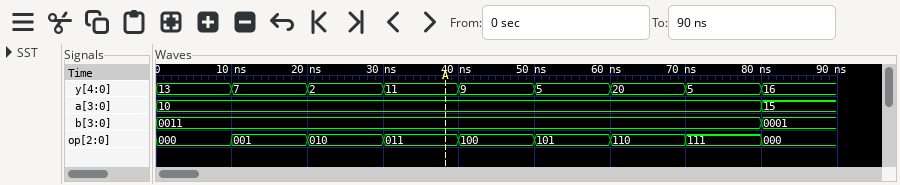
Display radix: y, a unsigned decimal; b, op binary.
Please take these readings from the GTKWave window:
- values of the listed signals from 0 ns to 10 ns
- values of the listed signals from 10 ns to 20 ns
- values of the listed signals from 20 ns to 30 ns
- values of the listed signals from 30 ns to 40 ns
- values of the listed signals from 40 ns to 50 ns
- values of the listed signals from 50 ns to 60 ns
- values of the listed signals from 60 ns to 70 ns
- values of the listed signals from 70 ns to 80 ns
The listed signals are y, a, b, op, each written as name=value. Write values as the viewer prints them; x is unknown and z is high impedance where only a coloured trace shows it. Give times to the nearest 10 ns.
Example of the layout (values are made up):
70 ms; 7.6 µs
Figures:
y=13, a=10, b=0011, op=000; y=7, a=10, b=0011, op=001; y=2, a=10, b=0011, op=010; y=11, a=10, b=0011, op=011; y=9, a=10, b=0011, op=100; y=5, a=10, b=0011, op=101; y=20, a=10, b=0011, op=110; y=5, a=10, b=0011, op=111
